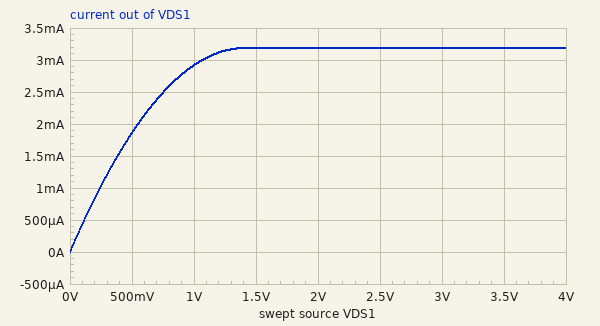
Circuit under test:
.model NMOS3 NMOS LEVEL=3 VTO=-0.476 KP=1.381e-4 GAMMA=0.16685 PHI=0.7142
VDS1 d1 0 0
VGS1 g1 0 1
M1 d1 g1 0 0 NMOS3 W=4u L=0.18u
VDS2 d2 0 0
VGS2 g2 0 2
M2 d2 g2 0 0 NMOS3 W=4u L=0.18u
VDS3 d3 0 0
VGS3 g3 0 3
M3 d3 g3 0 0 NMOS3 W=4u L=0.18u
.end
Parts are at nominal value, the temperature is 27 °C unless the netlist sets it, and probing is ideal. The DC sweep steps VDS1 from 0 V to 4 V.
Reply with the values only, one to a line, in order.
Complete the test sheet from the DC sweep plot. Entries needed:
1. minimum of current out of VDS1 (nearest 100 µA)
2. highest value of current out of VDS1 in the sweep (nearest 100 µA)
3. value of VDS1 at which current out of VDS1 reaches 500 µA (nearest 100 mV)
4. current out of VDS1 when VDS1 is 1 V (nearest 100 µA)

0 A
3.2 mA
100 mV
2.9 mA
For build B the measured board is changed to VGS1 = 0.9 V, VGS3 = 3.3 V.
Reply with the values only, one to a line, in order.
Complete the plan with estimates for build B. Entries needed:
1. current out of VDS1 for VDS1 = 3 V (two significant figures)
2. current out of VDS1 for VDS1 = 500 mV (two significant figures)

2.8 mA
1.7 mA
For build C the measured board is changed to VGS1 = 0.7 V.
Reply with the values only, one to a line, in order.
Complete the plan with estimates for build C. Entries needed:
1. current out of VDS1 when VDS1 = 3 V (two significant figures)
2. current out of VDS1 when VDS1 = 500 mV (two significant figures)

2.0 mA
1.4 mA
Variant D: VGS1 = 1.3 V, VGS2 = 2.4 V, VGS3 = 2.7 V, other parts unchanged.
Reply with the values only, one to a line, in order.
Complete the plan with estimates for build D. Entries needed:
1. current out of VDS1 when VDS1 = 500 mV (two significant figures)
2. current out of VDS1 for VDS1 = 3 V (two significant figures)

2.3 mA
4.6 mA
